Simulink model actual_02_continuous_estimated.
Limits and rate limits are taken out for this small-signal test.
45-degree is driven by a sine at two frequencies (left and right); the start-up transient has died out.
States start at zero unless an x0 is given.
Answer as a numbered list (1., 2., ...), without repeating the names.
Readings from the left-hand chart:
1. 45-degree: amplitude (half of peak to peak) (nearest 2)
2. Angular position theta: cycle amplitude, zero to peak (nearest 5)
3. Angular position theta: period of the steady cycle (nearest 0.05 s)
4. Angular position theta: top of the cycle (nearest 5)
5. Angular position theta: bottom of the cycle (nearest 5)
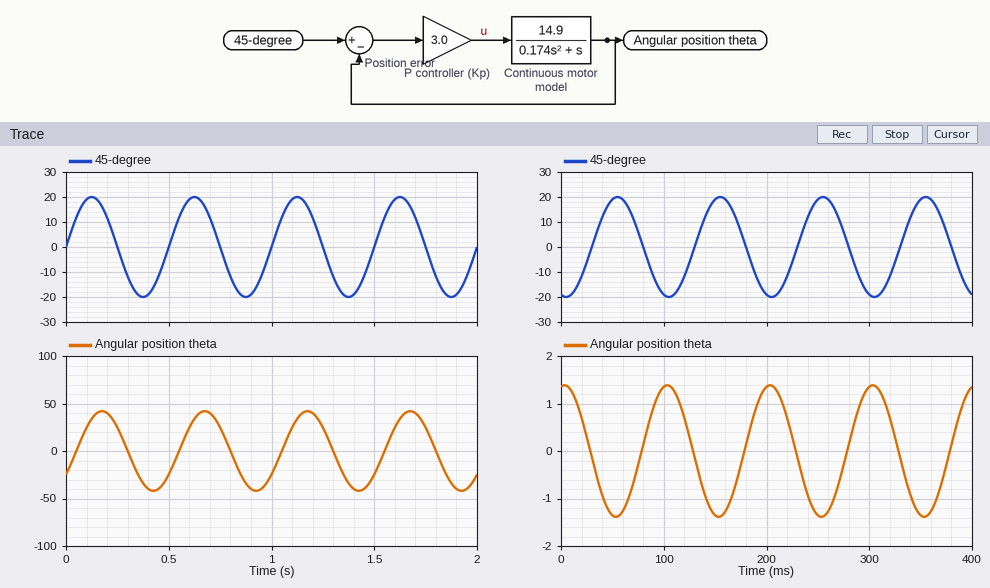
1. 20
2. 40
3. 0.50 s
4. 40
5. -40
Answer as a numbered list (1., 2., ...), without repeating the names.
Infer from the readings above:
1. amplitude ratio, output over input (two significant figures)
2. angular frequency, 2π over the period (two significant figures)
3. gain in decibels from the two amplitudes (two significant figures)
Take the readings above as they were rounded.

1. 2.0
2. 13 rad/s
3. 6.0 dB
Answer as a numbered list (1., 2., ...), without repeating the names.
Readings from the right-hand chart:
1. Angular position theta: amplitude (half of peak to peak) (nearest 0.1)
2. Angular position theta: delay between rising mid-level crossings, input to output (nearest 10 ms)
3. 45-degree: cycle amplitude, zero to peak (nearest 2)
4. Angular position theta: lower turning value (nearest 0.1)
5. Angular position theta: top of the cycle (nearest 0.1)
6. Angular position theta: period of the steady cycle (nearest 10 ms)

1. 1.4
2. 50 ms
3. 20
4. -1.4
5. 1.4
6. 100 ms
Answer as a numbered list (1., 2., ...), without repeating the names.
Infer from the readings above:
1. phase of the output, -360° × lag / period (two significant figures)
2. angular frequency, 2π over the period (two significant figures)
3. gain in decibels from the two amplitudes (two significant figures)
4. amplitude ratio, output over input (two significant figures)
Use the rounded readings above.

1. -180°
2. 0.063 rad/ms
3. -23 dB
4. 0.070
